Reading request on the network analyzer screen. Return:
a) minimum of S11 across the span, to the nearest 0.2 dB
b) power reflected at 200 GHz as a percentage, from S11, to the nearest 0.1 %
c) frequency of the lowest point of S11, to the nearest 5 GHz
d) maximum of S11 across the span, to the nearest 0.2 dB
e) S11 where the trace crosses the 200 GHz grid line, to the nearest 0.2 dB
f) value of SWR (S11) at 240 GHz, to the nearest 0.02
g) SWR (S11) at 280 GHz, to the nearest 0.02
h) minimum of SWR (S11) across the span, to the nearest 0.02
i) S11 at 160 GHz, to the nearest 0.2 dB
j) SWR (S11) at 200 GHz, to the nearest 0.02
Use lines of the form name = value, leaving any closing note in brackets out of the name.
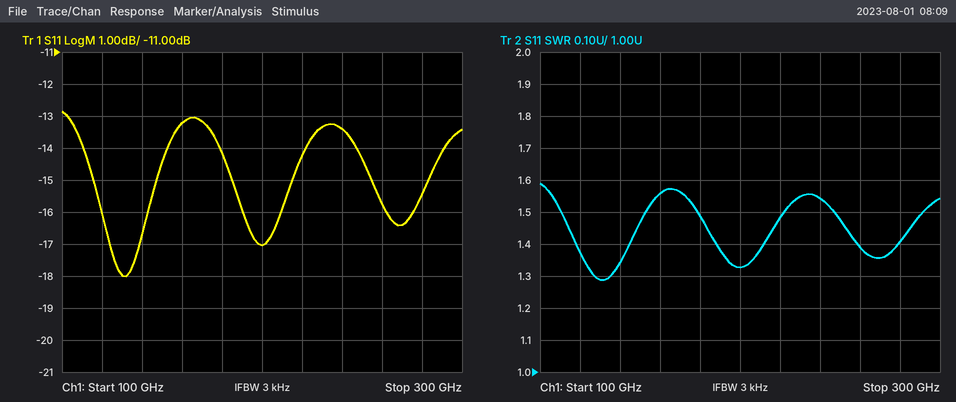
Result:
minimum of S11 across the span, to the nearest 0.2 dB = -18.0 dB
power reflected at 200 GHz as a percentage, from S11, to the nearest 0.1 % = 2.0 %
frequency of the lowest point of S11, to the nearest 5 GHz = 130 GHz
maximum of S11 across the span, to the nearest 0.2 dB = -12.8 dB
S11 where the trace crosses the 200 GHz grid line, to the nearest 0.2 dB = -17.0 dB
value of SWR (S11) at 240 GHz, to the nearest 0.02 = 1.54
SWR (S11) at 280 GHz, to the nearest 0.02 = 1.40
minimum of SWR (S11) across the span, to the nearest 0.02 = 1.28
S11 at 160 GHz, to the nearest 0.2 dB = -13.2 dB
SWR (S11) at 200 GHz, to the nearest 0.02 = 1.32
